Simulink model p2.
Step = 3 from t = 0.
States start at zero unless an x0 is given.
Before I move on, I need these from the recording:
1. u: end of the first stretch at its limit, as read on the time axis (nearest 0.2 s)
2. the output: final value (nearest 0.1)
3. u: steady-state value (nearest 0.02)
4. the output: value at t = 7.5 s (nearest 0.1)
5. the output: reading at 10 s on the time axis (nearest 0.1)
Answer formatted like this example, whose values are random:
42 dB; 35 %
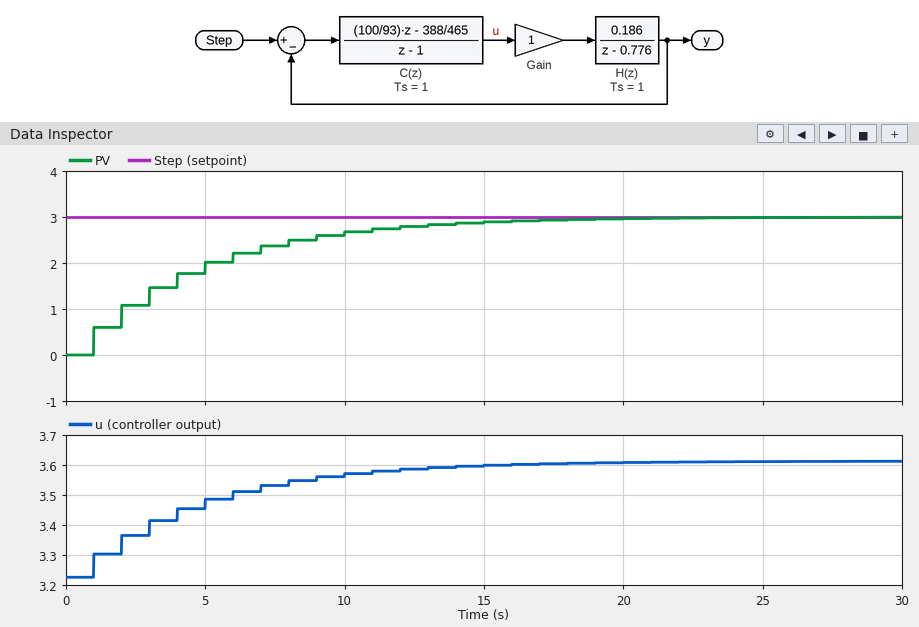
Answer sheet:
1.0 s; 3.0; 3.62; 2.4; 2.7
